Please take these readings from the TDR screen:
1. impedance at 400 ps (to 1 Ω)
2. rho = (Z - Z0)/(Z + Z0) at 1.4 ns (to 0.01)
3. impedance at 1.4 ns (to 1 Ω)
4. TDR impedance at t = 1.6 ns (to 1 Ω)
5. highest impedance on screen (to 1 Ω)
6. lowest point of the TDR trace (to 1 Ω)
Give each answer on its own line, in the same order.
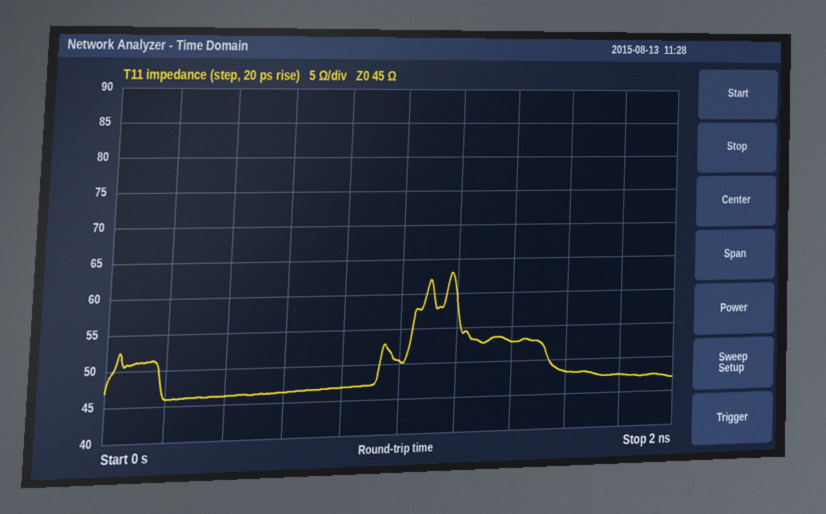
46 Ω
+0.08
53 Ω
48 Ω
63 Ω
46 Ω
